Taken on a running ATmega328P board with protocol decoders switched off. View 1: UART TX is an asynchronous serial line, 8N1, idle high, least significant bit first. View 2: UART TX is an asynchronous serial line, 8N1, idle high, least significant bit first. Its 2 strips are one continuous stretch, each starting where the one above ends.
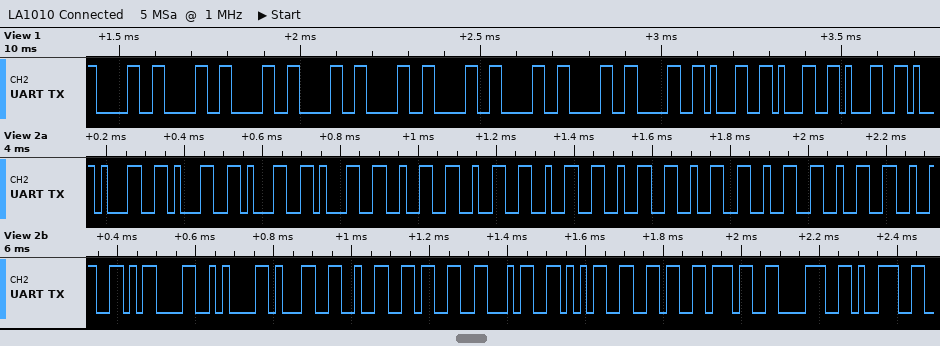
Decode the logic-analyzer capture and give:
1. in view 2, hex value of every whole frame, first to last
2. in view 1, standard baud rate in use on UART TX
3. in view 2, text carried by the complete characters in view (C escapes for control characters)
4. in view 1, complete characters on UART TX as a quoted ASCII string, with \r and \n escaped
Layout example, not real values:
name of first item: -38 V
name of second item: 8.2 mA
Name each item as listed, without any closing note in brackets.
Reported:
in view 2, hex value of every whole frame, first to last: 31 31 31 31 32 32 32 32 32 32 32 32 0D 0A 31 32 33 34 35 36 37 38 39
in view 1, standard baud rate in use on UART TX: 57600 baud
in view 2, text carried by the complete characters in view: "111122222222\r\n123456789"
in view 1, complete characters on UART TX as a quoted ASCII string, with \r and \n escaped: "000000000111"
